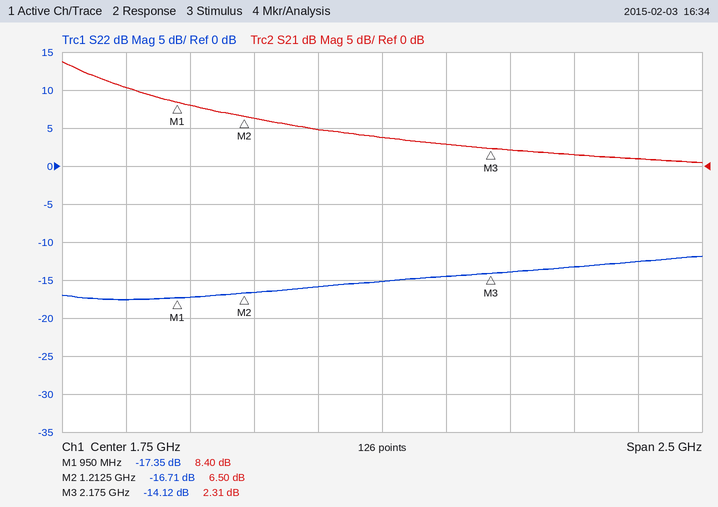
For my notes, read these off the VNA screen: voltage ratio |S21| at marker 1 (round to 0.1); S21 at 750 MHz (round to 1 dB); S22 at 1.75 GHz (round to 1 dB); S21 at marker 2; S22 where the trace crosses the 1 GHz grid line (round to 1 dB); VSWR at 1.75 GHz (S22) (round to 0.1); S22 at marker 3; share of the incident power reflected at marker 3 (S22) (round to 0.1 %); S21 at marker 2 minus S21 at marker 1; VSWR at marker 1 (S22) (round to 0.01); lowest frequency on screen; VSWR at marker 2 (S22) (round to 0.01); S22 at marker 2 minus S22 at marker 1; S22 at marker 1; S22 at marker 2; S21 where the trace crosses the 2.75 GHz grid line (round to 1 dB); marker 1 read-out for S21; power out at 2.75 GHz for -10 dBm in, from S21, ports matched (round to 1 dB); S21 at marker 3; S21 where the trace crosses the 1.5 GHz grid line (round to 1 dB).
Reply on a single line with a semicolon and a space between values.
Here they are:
2.6; 10 dB; -15 dB; 6.50 dB; -17 dB; 1.4; -14.12 dB; 3.9 %; -1.90 dB; 1.31; 500 MHz; 1.34; 0.64 dB; -17.35 dB; -16.71 dB; 1 dB; 8.40 dB; -9 dBm; 2.31 dB; 5 dB
